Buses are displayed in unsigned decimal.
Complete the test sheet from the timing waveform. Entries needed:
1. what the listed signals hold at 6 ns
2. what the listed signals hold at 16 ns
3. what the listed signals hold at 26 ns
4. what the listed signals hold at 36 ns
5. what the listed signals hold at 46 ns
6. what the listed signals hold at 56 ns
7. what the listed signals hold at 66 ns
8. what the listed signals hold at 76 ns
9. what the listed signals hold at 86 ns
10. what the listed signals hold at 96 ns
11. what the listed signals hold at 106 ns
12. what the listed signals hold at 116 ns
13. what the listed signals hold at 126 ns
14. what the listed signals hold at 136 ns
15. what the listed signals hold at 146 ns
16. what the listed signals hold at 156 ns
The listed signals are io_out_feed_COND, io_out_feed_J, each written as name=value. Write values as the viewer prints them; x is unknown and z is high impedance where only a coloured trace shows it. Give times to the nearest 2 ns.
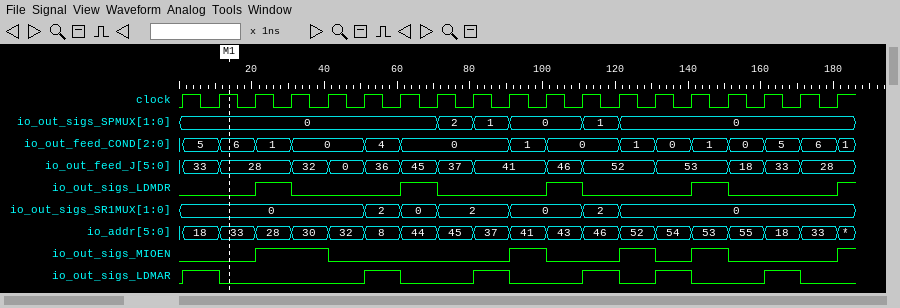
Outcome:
io_out_feed_COND=5, io_out_feed_J=33
io_out_feed_COND=6, io_out_feed_J=28
io_out_feed_COND=1, io_out_feed_J=28
io_out_feed_COND=0, io_out_feed_J=32
io_out_feed_COND=0, io_out_feed_J=0
io_out_feed_COND=4, io_out_feed_J=36
io_out_feed_COND=0, io_out_feed_J=45
io_out_feed_COND=0, io_out_feed_J=37
io_out_feed_COND=0, io_out_feed_J=41
io_out_feed_COND=1, io_out_feed_J=41
io_out_feed_COND=0, io_out_feed_J=46
io_out_feed_COND=0, io_out_feed_J=52
io_out_feed_COND=1, io_out_feed_J=52
io_out_feed_COND=0, io_out_feed_J=53
io_out_feed_COND=1, io_out_feed_J=53
io_out_feed_COND=0, io_out_feed_J=18
